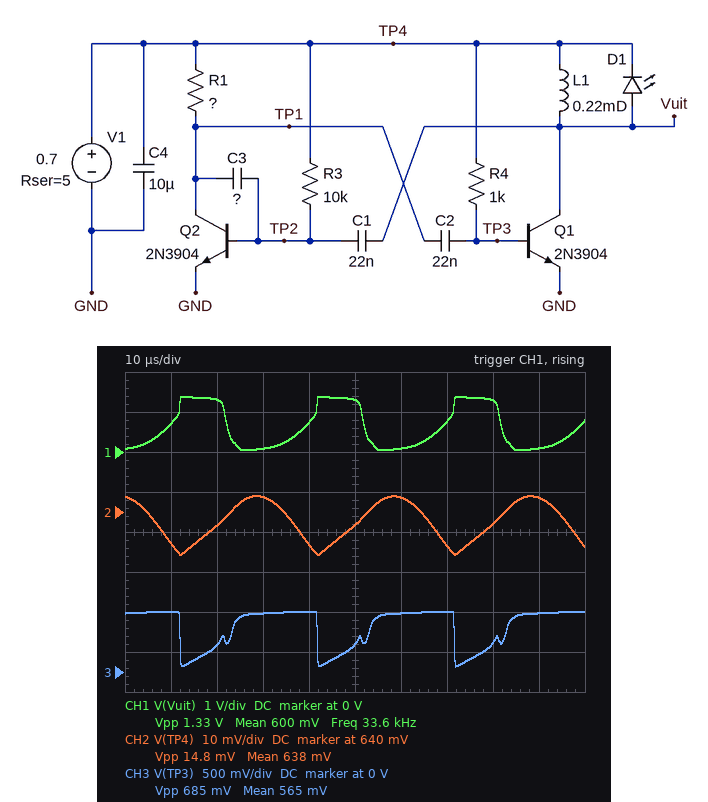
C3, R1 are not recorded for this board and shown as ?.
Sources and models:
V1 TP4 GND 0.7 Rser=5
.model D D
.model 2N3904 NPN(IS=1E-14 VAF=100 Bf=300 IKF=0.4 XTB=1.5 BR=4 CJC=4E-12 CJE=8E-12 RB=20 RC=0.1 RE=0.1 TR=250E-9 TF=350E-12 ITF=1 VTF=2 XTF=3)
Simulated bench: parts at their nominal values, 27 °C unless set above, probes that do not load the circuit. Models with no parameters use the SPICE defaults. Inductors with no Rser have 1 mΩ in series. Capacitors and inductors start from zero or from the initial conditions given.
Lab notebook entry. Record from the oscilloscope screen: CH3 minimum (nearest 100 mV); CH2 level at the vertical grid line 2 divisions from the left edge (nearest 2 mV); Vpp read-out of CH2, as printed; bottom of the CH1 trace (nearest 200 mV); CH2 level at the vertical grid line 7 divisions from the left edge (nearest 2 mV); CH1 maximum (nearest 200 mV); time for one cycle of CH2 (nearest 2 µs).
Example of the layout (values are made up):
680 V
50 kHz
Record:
100 mV
636 mV
14.8 mV
0 V
632 mV
1.4 V
30 µs
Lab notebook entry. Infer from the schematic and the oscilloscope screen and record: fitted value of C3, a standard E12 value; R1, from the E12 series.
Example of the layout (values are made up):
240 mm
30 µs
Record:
10 nF
150 Ω
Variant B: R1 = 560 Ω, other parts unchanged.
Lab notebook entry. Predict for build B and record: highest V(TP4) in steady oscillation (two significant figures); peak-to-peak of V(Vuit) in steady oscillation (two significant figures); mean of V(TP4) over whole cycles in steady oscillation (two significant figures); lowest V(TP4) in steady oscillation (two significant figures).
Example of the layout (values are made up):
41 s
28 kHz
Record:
630 mV
1.2 V
620 mV
600 mV
